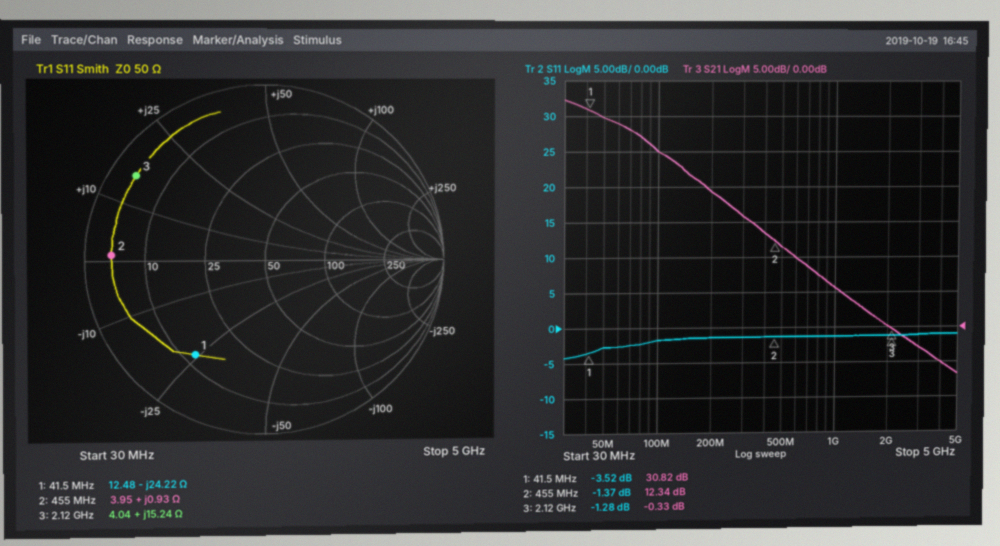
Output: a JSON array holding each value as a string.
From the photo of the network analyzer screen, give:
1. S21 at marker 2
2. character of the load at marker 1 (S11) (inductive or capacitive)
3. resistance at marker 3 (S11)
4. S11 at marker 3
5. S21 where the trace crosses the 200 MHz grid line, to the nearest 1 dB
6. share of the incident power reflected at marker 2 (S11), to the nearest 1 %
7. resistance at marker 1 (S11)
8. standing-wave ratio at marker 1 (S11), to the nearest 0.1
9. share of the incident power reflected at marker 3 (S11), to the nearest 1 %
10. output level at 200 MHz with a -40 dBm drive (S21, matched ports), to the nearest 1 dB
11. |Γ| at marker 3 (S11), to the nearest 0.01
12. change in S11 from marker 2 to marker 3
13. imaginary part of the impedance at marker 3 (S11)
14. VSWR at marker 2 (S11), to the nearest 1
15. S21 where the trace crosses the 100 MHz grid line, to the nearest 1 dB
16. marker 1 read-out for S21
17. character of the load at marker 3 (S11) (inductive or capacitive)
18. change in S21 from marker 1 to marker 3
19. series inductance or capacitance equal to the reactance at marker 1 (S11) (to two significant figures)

["12.34 dB", "capacitive", "4.04 Ω", "-1.28 dB", "19 dB", "73 %", "12.48 Ω", "5.0", "74 %", "-21 dBm", "0.86", "0.09 dB", "+15.24 Ω", "13", "25 dB", "30.82 dB", "inductive", "-31.15 dB", "160 pF"]
